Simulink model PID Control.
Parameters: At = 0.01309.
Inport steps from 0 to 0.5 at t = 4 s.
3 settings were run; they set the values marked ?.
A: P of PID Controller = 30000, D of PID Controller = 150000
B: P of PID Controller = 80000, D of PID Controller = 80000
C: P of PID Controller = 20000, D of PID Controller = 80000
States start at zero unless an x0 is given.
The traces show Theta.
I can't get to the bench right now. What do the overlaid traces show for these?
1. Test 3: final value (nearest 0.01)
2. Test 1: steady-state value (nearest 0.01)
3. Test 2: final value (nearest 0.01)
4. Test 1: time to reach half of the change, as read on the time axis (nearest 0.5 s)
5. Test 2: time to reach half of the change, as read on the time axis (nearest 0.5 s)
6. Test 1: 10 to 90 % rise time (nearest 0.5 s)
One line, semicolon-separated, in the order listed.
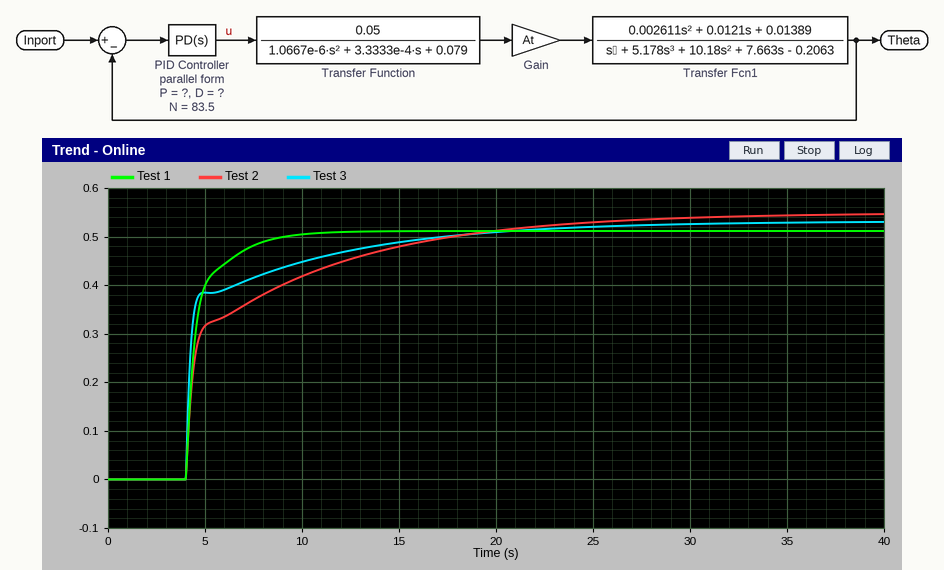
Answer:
0.53; 0.51; 0.55; 4.5 s; 4.5 s; 2.5 s
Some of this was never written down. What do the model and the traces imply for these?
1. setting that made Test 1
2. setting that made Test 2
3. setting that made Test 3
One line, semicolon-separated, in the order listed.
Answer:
B; C; A
